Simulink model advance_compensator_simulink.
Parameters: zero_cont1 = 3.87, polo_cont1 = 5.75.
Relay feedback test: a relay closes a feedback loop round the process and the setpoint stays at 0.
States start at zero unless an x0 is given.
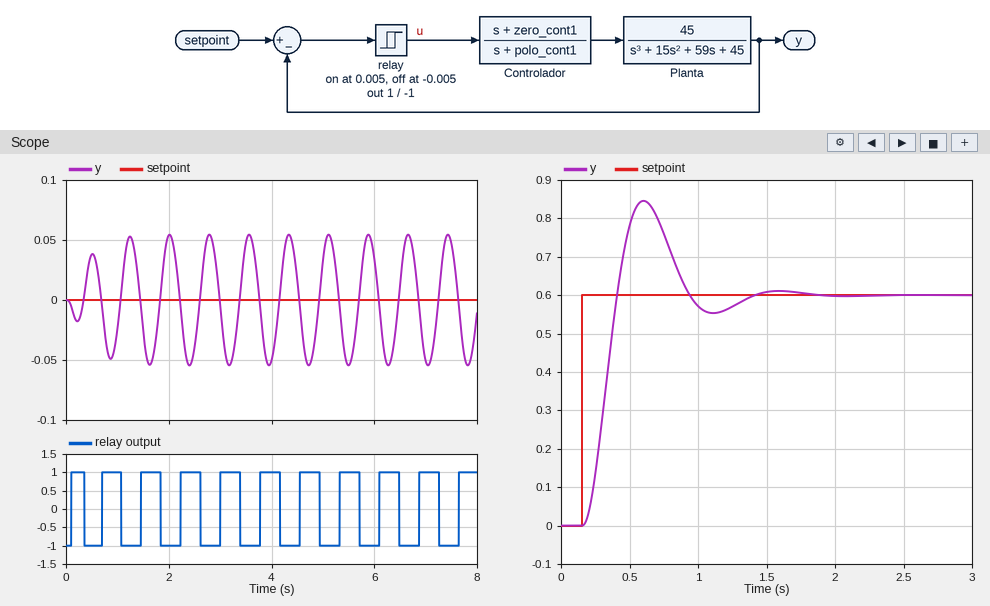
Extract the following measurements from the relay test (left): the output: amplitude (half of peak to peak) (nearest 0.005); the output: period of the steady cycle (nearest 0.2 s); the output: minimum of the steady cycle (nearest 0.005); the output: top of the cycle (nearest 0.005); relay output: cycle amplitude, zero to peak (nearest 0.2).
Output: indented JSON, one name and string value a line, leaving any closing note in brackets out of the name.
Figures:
{
  "the output: amplitude (half of peak to peak)": "0.055",
  "the output: period of the steady cycle": "0.8 s",
  "the output: minimum of the steady cycle": "-0.055",
  "the output: top of the cycle": "0.055",
  "relay output: cycle amplitude, zero to peak": "1.0"
}
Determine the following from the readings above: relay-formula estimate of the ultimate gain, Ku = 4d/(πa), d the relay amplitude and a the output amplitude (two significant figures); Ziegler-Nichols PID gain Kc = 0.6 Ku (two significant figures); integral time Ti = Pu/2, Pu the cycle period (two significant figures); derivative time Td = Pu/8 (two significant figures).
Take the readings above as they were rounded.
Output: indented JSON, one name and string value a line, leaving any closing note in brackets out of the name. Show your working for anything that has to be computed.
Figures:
{
  "relay-formula estimate of the ultimate gain, Ku = 4d/(πa), d the relay amplitude and a the output amplitude": "4 × 1 / (π × 0.055) = 23",
  "Ziegler-Nichols PID gain Kc = 0.6 Ku": "0.6 × 23 = 14",
  "integral time Ti = Pu/2, Pu the cycle period": "0.8 / 2 = 0.40 s",
  "derivative time Td = Pu/8": "0.8 / 8 = 0.10 s"
}
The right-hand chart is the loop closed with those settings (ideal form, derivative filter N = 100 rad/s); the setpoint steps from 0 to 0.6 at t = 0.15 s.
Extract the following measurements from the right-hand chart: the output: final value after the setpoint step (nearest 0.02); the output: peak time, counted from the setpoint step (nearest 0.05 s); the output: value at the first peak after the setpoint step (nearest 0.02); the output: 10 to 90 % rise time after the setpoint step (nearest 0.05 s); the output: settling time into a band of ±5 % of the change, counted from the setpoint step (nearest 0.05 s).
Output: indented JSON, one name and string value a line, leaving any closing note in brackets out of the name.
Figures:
{
  "the output: final value after the setpoint step": "0.60",
  "the output: peak time, counted from the setpoint step": "0.45 s",
  "the output: value at the first peak after the setpoint step": "0.84",
  "the output: 10 to 90 % rise time after the setpoint step": "0.15 s",
  "the output: settling time into a band of ±5 % of the change, counted from the setpoint step": "1.10 s"
}
